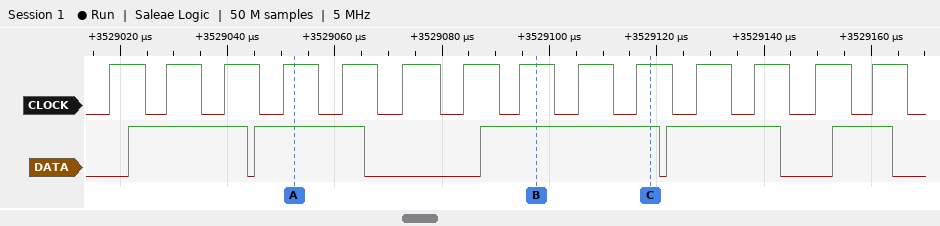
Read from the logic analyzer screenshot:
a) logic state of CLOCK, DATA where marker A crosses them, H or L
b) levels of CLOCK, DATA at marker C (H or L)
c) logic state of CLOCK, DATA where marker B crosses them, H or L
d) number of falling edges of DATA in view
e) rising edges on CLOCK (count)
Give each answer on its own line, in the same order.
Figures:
CLOCK=H, DATA=H
CLOCK=H, DATA=H
CLOCK=H, DATA=H
5
14
